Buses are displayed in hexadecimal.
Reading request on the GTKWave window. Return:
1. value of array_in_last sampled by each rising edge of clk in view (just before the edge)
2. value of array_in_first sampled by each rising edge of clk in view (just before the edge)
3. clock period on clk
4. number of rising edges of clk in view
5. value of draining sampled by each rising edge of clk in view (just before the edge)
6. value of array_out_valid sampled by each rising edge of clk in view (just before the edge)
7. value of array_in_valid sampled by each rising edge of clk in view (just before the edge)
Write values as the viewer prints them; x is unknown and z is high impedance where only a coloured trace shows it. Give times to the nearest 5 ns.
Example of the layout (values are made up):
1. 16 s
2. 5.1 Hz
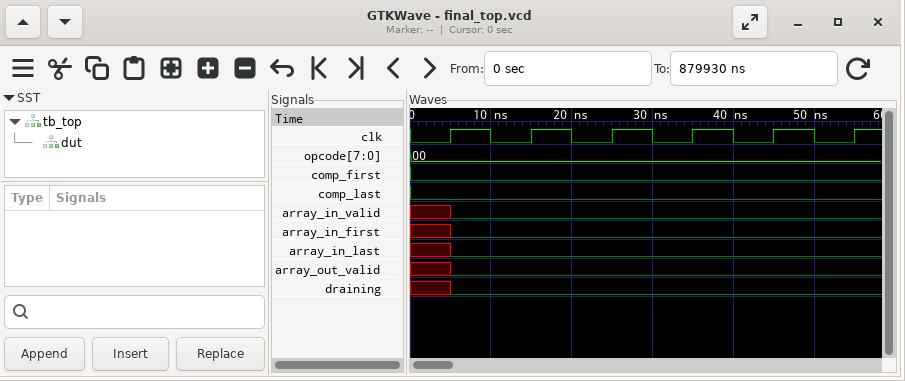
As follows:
1. x 0 0 0 0 0
2. x 0 0 0 0 0
3. 10 ns
4. 6
5. x 0 0 0 0 0
6. x 0 0 0 0 0
7. x 0 0 0 0 0
